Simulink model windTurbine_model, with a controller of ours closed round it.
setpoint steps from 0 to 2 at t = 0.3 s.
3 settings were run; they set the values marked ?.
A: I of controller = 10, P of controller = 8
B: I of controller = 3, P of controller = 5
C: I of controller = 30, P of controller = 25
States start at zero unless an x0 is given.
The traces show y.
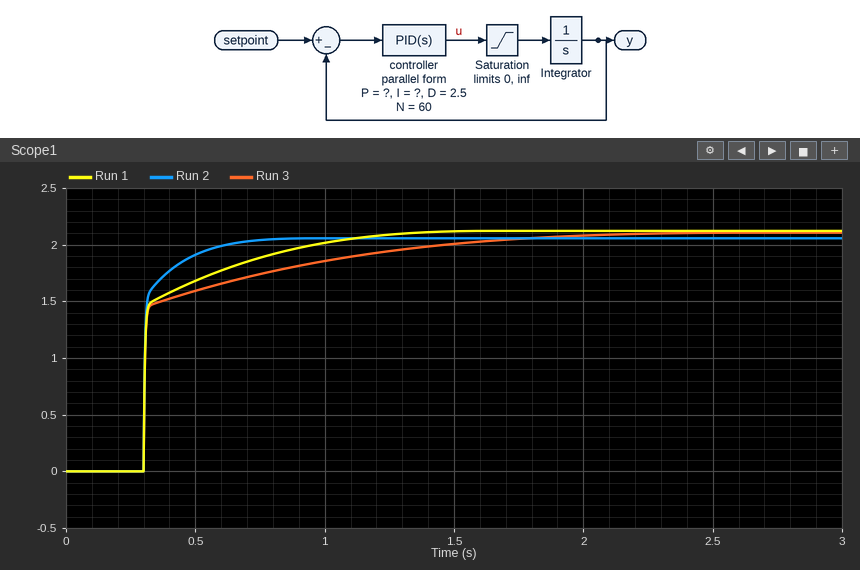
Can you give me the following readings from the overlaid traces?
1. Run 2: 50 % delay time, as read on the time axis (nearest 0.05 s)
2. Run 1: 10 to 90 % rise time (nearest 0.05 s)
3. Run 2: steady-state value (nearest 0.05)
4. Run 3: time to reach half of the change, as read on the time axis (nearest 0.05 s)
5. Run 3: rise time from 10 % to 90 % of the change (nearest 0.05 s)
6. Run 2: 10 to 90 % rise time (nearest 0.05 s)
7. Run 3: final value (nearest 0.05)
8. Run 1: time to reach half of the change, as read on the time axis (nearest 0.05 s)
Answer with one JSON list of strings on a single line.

["0.30 s", "0.50 s", "2.05", "0.30 s", "0.80 s", "0.15 s", "2.10", "0.30 s"]
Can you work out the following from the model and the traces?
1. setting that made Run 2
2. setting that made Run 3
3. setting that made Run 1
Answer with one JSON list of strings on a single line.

["C", "B", "A"]
